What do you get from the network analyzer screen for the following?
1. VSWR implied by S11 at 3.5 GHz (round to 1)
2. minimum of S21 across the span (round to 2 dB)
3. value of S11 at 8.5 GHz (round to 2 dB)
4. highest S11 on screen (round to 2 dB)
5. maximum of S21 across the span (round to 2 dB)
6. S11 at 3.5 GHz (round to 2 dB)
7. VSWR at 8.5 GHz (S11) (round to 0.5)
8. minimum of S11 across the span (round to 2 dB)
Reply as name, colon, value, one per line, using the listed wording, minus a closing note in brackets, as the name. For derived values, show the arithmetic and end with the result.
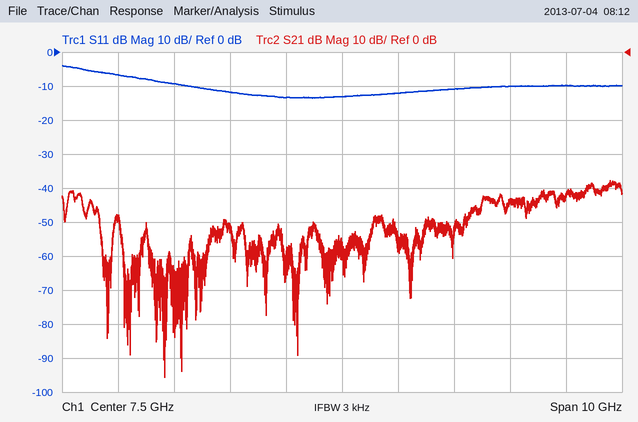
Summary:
VSWR implied by S11 at 3.5 GHz: |Γ| = 10^(-6/20) = 0.5012; VSWR = (1 + 0.5012)/(1 − 0.5012) ≈ 3
minimum of S21 across the span: -96 dB
value of S11 at 8.5 GHz: -12 dB
highest S11 on screen: -4 dB
maximum of S21 across the span: -38 dB
S11 at 3.5 GHz: -6 dB
VSWR at 8.5 GHz (S11): |Γ| = 10^(-12/20) = 0.2512; VSWR = (1 + 0.2512)/(1 − 0.2512) ≈ 1.67, so 1.5 to the nearest 0.5
minimum of S11 across the span: -14 dB
